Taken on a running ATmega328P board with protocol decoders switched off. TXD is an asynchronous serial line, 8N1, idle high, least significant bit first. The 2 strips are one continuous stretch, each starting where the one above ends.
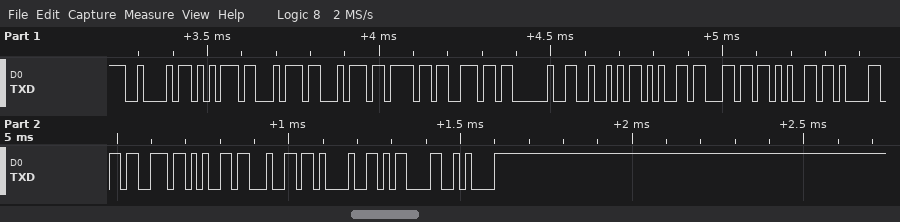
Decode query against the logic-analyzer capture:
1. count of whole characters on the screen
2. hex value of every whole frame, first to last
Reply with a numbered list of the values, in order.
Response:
1. 18
2. 42 75 74 74 6F 6E 20 52 65 6C 65 61 73 65 64 21 0D 0A
